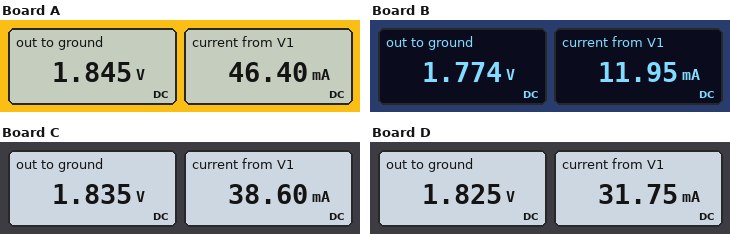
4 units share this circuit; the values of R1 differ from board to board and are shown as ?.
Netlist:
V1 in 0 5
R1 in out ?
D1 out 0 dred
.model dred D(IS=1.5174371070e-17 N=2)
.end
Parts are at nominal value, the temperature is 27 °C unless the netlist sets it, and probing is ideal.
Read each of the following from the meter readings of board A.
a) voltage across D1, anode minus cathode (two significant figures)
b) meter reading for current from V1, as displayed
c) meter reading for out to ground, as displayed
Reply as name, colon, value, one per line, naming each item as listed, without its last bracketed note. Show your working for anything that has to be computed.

voltage across D1, anode minus cathode: 1.845 V = 1.8 V
meter reading for current from V1, as displayed: 46.40 mA
meter reading for out to ground, as displayed: 1.845 V
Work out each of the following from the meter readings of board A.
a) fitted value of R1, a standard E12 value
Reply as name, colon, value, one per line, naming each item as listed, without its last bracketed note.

fitted value of R1, a standard E12 value: 68 Ω
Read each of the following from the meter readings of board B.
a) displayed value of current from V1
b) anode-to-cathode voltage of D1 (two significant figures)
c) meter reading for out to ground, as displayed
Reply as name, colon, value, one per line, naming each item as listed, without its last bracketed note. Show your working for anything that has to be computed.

displayed value of current from V1: 11.95 mA
anode-to-cathode voltage of D1: 1.774 V = 1.8 V
meter reading for out to ground, as displayed: 1.774 V
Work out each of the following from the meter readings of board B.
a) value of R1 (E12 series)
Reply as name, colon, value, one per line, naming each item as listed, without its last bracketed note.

value of R1: 270 Ω
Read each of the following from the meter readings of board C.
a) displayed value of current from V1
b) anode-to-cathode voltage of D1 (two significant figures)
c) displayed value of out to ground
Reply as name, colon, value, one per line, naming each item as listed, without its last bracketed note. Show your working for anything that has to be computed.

displayed value of current from V1: 38.60 mA
anode-to-cathode voltage of D1: 1.835 V = 1.8 V
displayed value of out to ground: 1.835 V
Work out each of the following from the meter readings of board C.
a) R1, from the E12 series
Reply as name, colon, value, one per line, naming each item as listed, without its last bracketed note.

R1, from the E12 series: 82 Ω
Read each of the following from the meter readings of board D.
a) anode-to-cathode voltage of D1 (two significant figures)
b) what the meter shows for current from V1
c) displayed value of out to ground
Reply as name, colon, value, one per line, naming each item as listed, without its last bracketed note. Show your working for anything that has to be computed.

anode-to-cathode voltage of D1: 1.825 V = 1.8 V
what the meter shows for current from V1: 31.75 mA
displayed value of out to ground: 1.825 V
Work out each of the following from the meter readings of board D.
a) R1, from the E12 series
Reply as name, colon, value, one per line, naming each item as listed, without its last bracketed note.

R1, from the E12 series: 100 Ω
